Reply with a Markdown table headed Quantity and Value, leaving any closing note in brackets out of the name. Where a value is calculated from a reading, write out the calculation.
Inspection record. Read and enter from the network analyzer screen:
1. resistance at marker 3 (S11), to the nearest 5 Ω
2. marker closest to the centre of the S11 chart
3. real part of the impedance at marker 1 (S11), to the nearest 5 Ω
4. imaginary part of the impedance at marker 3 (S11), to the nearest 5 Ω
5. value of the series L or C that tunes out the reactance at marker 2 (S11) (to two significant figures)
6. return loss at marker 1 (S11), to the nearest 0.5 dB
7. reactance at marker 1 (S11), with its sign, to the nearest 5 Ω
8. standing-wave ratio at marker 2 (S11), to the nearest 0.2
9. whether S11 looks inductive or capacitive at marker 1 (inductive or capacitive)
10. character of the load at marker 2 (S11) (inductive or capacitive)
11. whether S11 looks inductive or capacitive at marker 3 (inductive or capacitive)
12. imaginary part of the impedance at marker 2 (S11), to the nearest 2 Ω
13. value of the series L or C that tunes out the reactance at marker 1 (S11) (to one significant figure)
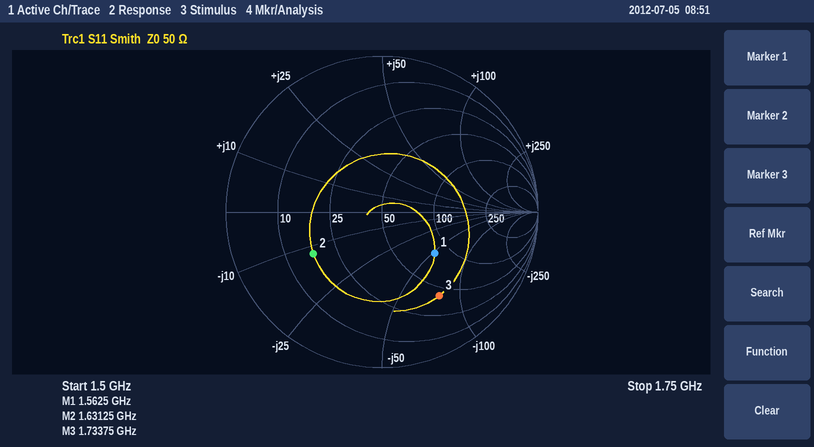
| Quantity | Value |
|---|---|
| resistance at marker 3 (S11), to the nearest 5 Ω | 40 Ω |
| marker closest to the centre of the S11 chart | marker 1 |
| real part of the impedance at marker 1 (S11), to the nearest 5 Ω | 80 Ω |
| imaginary part of the impedance at marker 3 (S11), to the nearest 5 Ω | -80 Ω |
| value of the series L or C that tunes out the reactance at marker 2 (S11) | L = 12 Ω/(2π × 1.63125 GHz) ≈ 1.2 nH |
| return loss at marker 1 (S11), to the nearest 0.5 dB | 7.5 dB |
| reactance at marker 1 (S11), with its sign, to the nearest 5 Ω | -50 Ω |
| standing-wave ratio at marker 2 (S11), to the nearest 0.2 | 3.2 |
| whether S11 looks inductive or capacitive at marker 1 | capacitive |
| character of the load at marker 2 (S11) | capacitive |
| whether S11 looks inductive or capacitive at marker 3 | capacitive |
| imaginary part of the impedance at marker 2 (S11), to the nearest 2 Ω | -12 Ω |
| value of the series L or C that tunes out the reactance at marker 1 (S11) | L = 50 Ω/(2π × 1.5625 GHz) ≈ 5 nH |
